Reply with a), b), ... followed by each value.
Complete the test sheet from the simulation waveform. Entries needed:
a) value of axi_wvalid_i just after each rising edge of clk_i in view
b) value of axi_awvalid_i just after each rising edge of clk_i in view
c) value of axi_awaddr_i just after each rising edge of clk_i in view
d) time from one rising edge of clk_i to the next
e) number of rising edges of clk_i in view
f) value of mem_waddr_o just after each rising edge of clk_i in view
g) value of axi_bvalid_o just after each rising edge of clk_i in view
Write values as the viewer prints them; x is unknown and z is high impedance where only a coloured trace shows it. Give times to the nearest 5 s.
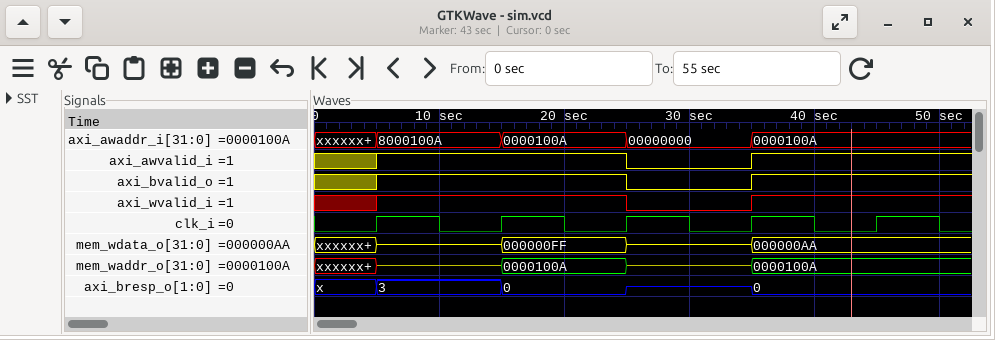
a) 1 1 0 1 1
b) 1 1 0 1 1
c) 8000100A, 0000100A, 00000000, 0000100A, 0000100A
d) 10 s
e) 5
f) z, 0000100A, z, 0000100A, 0000100A
g) 1 1 0 1 1
